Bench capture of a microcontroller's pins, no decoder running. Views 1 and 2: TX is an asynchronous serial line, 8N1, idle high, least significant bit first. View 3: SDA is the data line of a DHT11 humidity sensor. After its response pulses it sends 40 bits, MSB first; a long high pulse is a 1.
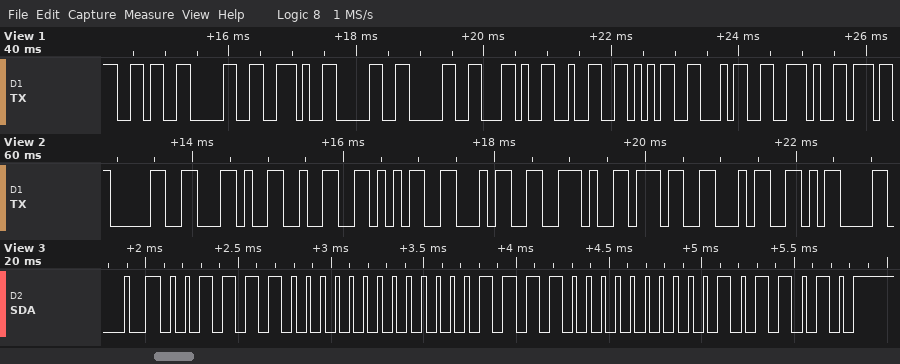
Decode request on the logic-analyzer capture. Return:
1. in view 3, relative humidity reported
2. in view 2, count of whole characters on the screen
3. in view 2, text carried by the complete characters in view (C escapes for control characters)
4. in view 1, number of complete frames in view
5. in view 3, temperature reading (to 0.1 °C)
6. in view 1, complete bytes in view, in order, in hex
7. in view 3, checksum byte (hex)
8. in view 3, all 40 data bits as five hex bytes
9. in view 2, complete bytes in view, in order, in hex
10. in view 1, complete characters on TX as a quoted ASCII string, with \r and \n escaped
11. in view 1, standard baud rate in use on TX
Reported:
60 %
9
"0,254.74\r"
10
30.0 °C
36 30 2E 30 30 2C 32 35 34 2E
0x5A
3C 00 1E 00 5A
0x30 0x2C 0x32 0x35 0x34 0x2E 0x37 0x34 0x0D
"60.00,254."
9600 baud
